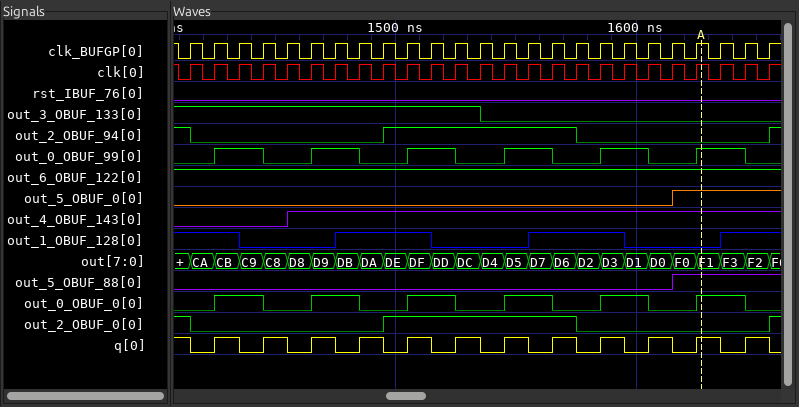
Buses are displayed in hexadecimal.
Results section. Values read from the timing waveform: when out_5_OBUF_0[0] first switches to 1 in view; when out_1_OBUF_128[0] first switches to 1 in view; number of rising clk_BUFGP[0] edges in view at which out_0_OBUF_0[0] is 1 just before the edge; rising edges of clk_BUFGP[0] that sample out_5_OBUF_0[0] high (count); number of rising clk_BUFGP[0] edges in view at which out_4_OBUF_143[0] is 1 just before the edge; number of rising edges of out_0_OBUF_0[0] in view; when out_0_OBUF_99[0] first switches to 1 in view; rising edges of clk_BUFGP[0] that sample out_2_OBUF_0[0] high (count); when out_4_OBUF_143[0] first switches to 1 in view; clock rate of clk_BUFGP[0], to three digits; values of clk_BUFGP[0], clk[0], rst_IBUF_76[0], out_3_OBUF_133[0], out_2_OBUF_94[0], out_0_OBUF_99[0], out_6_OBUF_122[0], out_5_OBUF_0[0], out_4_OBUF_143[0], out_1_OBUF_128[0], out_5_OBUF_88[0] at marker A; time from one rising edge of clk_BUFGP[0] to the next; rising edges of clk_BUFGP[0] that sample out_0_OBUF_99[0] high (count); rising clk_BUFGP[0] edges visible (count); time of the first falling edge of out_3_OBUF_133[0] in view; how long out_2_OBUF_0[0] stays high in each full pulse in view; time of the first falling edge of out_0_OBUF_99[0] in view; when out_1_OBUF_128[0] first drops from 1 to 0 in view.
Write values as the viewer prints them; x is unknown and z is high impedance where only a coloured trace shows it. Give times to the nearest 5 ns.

1615 ns
1475 ns
12
4
20
6
1425 ns
9
1455 ns
100 MHz
clk_BUFGP[0]=1, clk[0]=1, rst_IBUF_76[0]=0, out_3_OBUF_133[0]=0, out_2_OBUF_94[0]=0, out_0_OBUF_99[0]=1, out_6_OBUF_122[0]=1, out_5_OBUF_0[0]=1, out_4_OBUF_143[0]=1, out_1_OBUF_128[0]=0, out_5_OBUF_88[0]=1
10 ns
12
25
1535 ns
80 ns
1445 ns
1435 ns
